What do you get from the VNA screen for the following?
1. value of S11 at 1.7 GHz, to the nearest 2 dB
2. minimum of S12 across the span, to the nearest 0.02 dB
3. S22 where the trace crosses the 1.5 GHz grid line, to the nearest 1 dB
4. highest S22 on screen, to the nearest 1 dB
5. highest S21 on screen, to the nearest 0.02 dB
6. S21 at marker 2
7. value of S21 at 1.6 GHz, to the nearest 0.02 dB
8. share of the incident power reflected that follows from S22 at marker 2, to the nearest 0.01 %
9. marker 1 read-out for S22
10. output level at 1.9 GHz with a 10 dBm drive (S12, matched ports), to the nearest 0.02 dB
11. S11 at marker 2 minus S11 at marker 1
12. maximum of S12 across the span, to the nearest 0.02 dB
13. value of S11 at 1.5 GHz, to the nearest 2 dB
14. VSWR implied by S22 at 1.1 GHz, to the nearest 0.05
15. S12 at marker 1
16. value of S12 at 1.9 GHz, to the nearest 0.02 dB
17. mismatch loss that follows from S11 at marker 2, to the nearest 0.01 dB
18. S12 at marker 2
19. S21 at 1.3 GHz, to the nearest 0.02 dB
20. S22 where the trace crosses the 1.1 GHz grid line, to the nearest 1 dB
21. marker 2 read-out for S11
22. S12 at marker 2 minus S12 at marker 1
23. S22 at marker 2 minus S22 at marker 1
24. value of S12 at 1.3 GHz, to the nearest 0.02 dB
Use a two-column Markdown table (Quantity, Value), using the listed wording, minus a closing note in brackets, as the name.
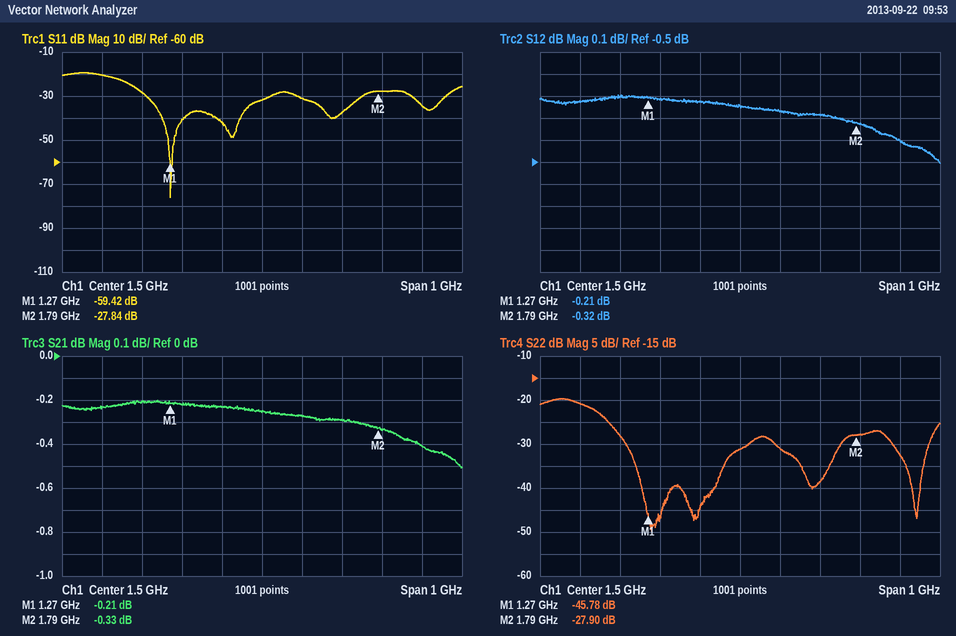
| Quantity | Value |
|---|---|
| value of S11 at 1.7 GHz, to the nearest 2 dB | -38 dB |
| minimum of S12 across the span, to the nearest 0.02 dB | -0.50 dB |
| S22 where the trace crosses the 1.5 GHz grid line, to the nearest 1 dB | -31 dB |
| highest S22 on screen, to the nearest 1 dB | -20 dB |
| highest S21 on screen, to the nearest 0.02 dB | -0.20 dB |
| S21 at marker 2 | -0.33 dB |
| value of S21 at 1.6 GHz, to the nearest 0.02 dB | -0.28 dB |
| share of the incident power reflected that follows from S22 at marker 2, to the nearest 0.01 % | 0.16 % |
| marker 1 read-out for S22 | -45.78 dB |
| output level at 1.9 GHz with a 10 dBm drive (S12, matched ports), to the nearest 0.02 dB | 9.60 dBm |
| S11 at marker 2 minus S11 at marker 1 | 31.58 dB |
| maximum of S12 across the span, to the nearest 0.02 dB | -0.20 dB |
| value of S11 at 1.5 GHz, to the nearest 2 dB | -32 dB |
| VSWR implied by S22 at 1.1 GHz, to the nearest 0.05 | 1.20 |
| S12 at marker 1 | -0.21 dB |
| value of S12 at 1.9 GHz, to the nearest 0.02 dB | -0.40 dB |
| mismatch loss that follows from S11 at marker 2, to the nearest 0.01 dB | 0.01 dB |
| S12 at marker 2 | -0.32 dB |
| S21 at 1.3 GHz, to the nearest 0.02 dB | -0.22 dB |
| S22 where the trace crosses the 1.1 GHz grid line, to the nearest 1 dB | -21 dB |
| marker 2 read-out for S11 | -27.84 dB |
| S12 at marker 2 minus S12 at marker 1 | -0.11 dB |
| S22 at marker 2 minus S22 at marker 1 | 17.88 dB |
| value of S12 at 1.3 GHz, to the nearest 0.02 dB | -0.22 dB |
